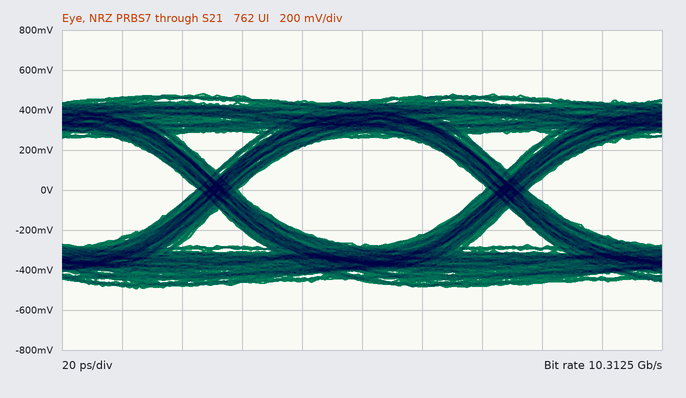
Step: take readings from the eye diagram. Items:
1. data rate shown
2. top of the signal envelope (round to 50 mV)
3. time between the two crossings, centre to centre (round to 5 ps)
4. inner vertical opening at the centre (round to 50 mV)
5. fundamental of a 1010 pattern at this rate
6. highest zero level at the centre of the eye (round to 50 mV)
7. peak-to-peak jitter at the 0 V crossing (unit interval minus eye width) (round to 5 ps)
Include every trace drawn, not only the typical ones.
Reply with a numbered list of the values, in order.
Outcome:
1. 10.3125 Gb/s
2. 500 mV
3. 95 ps
4. 550 mV
5. 5.15625 GHz
6. -300 mV
7. 15 ps
